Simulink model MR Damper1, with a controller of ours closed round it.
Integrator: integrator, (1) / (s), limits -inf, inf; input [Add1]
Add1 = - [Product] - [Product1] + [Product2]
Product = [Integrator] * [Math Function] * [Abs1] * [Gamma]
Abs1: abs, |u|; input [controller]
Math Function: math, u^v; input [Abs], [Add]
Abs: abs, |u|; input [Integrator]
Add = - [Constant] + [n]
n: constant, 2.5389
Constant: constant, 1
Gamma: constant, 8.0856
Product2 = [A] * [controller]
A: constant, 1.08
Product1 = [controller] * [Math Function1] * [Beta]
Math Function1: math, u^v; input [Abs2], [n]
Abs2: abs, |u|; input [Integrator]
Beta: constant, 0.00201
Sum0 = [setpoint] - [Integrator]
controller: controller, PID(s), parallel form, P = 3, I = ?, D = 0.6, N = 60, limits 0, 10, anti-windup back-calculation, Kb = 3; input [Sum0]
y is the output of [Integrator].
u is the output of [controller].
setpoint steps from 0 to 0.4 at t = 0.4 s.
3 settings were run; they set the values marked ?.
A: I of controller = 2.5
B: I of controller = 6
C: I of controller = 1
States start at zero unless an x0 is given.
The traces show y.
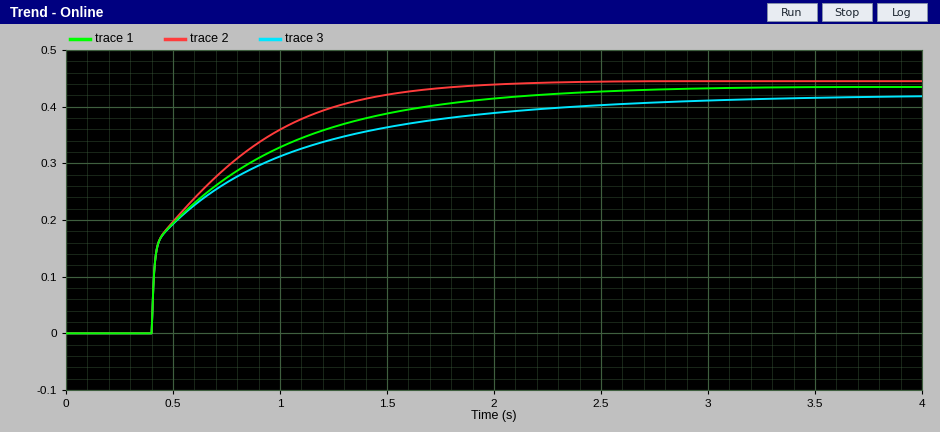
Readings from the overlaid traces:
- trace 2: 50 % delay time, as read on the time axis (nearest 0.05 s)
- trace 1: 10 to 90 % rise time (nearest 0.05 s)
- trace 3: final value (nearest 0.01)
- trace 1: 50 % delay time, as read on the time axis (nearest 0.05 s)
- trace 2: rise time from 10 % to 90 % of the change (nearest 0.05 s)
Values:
0.55 s
1.15 s
0.42
0.55 s
0.85 s
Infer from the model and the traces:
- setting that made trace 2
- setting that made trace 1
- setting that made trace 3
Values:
B
A
C
